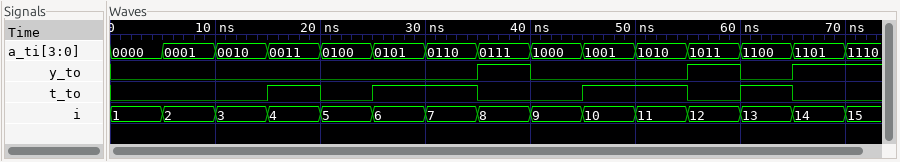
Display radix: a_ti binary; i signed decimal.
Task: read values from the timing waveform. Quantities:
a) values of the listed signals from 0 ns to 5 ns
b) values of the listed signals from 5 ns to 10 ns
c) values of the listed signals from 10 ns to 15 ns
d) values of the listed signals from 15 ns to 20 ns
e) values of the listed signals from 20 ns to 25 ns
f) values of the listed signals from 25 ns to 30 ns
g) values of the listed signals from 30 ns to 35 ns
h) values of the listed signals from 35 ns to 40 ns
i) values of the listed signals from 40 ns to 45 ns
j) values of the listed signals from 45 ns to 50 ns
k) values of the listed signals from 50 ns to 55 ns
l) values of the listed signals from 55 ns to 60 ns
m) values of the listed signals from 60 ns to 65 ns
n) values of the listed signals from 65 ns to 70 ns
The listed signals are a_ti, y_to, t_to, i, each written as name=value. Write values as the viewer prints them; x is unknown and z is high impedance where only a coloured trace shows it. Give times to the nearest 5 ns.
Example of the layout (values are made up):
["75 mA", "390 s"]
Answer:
["a_ti=0000, y_to=0, t_to=0, i=1", "a_ti=0001, y_to=0, t_to=0, i=2", "a_ti=0010, y_to=0, t_to=0, i=3", "a_ti=0011, y_to=0, t_to=1, i=4", "a_ti=0100, y_to=0, t_to=0, i=5", "a_ti=0101, y_to=0, t_to=1, i=6", "a_ti=0110, y_to=0, t_to=1, i=7", "a_ti=0111, y_to=1, t_to=0, i=8", "a_ti=1000, y_to=0, t_to=0, i=9", "a_ti=1001, y_to=0, t_to=1, i=10", "a_ti=1010, y_to=0, t_to=1, i=11", "a_ti=1011, y_to=1, t_to=0, i=12", "a_ti=1100, y_to=0, t_to=1, i=13", "a_ti=1101, y_to=1, t_to=0, i=14"]
